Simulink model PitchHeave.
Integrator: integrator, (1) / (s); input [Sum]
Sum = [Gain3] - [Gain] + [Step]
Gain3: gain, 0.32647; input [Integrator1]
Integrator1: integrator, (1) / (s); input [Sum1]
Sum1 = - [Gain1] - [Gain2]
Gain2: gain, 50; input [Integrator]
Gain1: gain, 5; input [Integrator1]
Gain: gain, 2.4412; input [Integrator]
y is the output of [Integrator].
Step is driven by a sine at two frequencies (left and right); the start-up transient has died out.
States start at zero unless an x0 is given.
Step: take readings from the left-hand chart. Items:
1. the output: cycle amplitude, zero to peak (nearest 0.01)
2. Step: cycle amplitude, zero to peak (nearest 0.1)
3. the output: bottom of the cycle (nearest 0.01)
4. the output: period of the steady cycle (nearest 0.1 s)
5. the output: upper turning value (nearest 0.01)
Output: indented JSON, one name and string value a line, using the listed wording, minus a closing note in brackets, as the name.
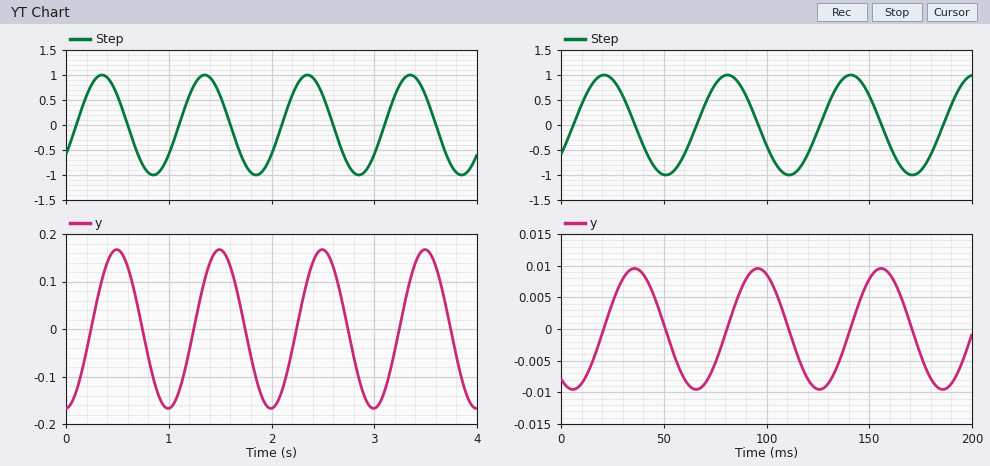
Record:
{
  "the output: cycle amplitude, zero to peak": "0.17",
  "Step: cycle amplitude, zero to peak": "1.0",
  "the output: bottom of the cycle": "-0.17",
  "the output: period of the steady cycle": "1.0 s",
  "the output: upper turning value": "0.17"
}
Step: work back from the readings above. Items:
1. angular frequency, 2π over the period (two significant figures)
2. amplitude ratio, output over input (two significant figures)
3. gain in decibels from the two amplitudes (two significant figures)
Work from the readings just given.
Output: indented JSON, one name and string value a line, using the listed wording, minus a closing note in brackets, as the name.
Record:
{
  "angular frequency, 2π over the period": "6.3 rad/s",
  "amplitude ratio, output over input": "0.17",
  "gain in decibels from the two amplitudes": "-15 dB"
}
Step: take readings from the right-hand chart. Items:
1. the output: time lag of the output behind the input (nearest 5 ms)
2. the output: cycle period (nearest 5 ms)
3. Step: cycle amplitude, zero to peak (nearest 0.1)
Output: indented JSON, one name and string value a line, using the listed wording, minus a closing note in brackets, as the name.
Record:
{
  "the output: time lag of the output behind the input": "15 ms",
  "the output: cycle period": "60 ms",
  "Step: cycle amplitude, zero to peak": "1.0"
}
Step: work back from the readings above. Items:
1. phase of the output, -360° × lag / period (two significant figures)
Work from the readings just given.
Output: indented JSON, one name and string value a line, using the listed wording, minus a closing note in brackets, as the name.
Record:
{
  "phase of the output, -360° × lag / period": "-90°"
}
